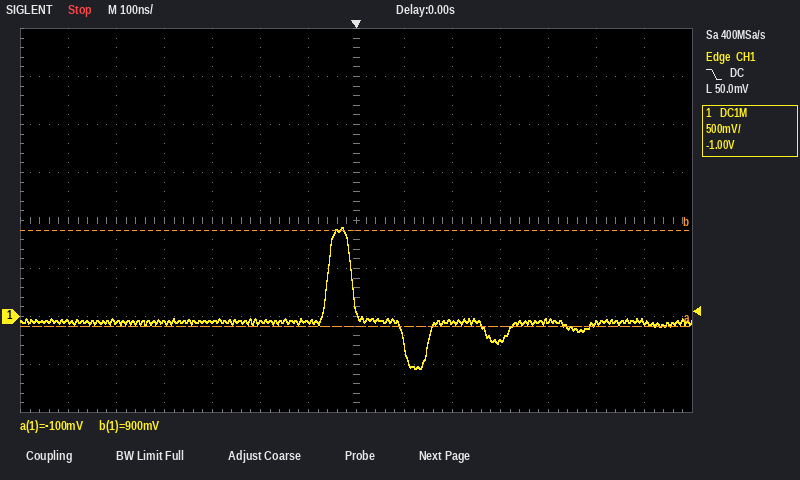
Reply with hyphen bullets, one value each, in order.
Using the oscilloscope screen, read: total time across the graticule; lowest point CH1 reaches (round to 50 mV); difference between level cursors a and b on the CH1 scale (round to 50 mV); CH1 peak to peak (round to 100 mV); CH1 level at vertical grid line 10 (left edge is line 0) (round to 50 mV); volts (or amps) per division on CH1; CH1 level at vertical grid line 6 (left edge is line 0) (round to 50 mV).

- 1.4 µs
- -550 mV
- 1.00 V
- 1.50 V
- -250 mV
- 500 mV
- -50 mV
